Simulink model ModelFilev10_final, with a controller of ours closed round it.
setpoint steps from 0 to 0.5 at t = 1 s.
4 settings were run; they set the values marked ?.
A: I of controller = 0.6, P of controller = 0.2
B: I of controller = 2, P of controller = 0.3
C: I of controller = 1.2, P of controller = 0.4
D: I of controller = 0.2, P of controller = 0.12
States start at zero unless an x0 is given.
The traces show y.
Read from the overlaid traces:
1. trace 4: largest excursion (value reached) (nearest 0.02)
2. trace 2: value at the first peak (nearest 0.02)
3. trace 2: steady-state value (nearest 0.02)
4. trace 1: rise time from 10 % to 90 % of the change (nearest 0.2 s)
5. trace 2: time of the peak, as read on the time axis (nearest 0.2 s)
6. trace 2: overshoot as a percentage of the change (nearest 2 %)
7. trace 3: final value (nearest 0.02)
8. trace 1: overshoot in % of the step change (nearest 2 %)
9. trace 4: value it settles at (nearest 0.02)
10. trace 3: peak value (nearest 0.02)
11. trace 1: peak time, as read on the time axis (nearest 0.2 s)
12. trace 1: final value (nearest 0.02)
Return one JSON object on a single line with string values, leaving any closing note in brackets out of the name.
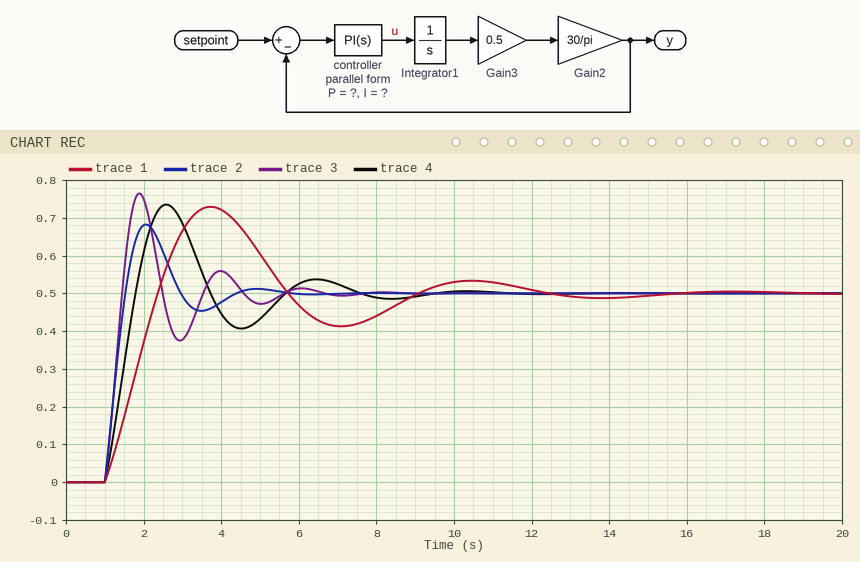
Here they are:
{"trace 4: largest excursion (value reached)": "0.74", "trace 2: value at the first peak": "0.68", "trace 2: steady-state value": "0.50", "trace 1: rise time from 10 % to 90 % of the change": "1.0 s", "trace 2: time of the peak, as read on the time axis": "2.0 s", "trace 2: overshoot as a percentage of the change": "36 %", "trace 3: final value": "0.50", "trace 1: overshoot in % of the step change": "46 %", "trace 4: value it settles at": "0.50", "trace 3: peak value": "0.76", "trace 1: peak time, as read on the time axis": "3.8 s", "trace 1: final value": "0.50"}
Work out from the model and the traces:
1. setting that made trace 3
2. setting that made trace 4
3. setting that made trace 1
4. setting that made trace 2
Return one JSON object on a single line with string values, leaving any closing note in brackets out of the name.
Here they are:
{"setting that made trace 3": "B", "setting that made trace 4": "A", "setting that made trace 1": "D", "setting that made trace 2": "C"}
